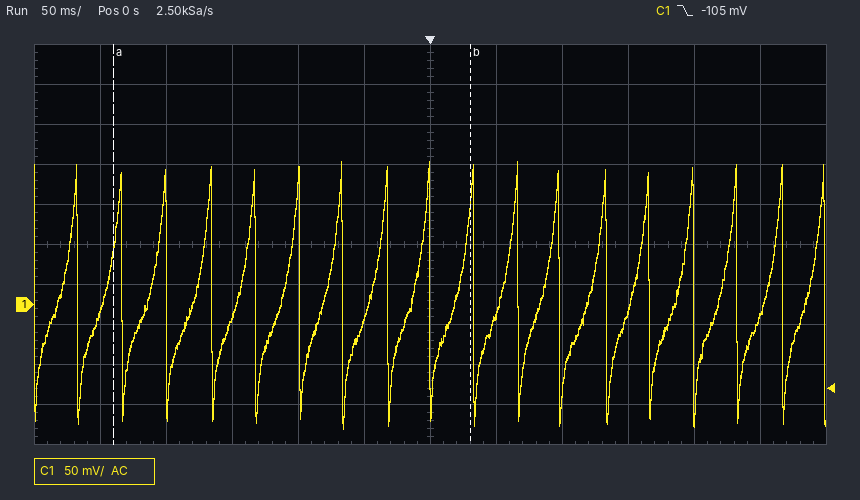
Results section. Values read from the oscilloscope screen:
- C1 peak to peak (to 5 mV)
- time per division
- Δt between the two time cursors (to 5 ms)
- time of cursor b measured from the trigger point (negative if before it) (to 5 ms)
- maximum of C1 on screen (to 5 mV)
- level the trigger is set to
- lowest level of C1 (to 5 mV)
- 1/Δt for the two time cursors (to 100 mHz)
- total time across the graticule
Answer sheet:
335 mV
50 ms
270 ms
+30 ms
180 mV
-105 mV
-155 mV
3.7 Hz
600 ms
